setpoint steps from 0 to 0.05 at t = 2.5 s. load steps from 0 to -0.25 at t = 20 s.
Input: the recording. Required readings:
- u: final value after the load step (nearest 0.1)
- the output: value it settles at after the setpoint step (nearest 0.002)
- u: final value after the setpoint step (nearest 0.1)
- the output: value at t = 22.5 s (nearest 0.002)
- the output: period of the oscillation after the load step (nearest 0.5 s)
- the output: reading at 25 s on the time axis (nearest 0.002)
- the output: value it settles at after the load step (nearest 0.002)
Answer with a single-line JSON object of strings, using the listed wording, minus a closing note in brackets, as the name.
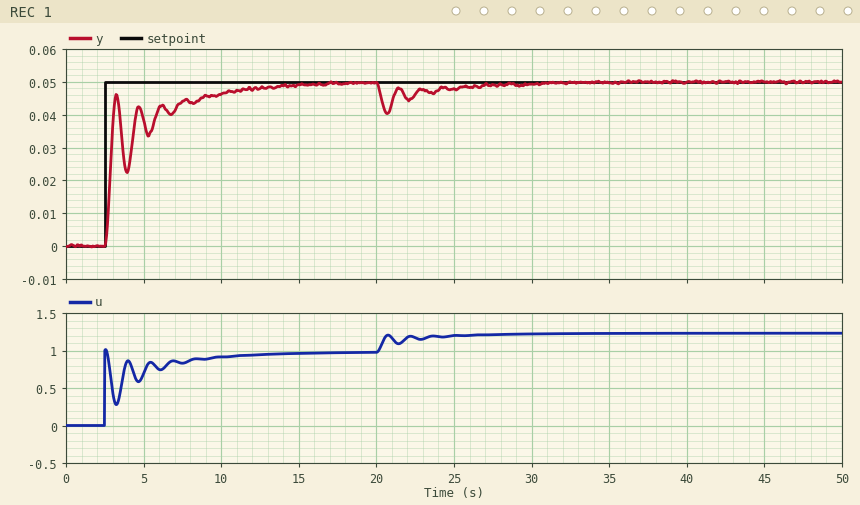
{"u: final value after the load step": "1.2", "the output: value it settles at after the setpoint step": "0.050", "u: final value after the setpoint step": "1.0", "the output: value at t = 22.5 s": "0.046", "the output: period of the oscillation after the load step": "1.5 s", "the output: reading at 25 s on the time axis": "0.048", "the output: value it settles at after the load step": "0.050"}
